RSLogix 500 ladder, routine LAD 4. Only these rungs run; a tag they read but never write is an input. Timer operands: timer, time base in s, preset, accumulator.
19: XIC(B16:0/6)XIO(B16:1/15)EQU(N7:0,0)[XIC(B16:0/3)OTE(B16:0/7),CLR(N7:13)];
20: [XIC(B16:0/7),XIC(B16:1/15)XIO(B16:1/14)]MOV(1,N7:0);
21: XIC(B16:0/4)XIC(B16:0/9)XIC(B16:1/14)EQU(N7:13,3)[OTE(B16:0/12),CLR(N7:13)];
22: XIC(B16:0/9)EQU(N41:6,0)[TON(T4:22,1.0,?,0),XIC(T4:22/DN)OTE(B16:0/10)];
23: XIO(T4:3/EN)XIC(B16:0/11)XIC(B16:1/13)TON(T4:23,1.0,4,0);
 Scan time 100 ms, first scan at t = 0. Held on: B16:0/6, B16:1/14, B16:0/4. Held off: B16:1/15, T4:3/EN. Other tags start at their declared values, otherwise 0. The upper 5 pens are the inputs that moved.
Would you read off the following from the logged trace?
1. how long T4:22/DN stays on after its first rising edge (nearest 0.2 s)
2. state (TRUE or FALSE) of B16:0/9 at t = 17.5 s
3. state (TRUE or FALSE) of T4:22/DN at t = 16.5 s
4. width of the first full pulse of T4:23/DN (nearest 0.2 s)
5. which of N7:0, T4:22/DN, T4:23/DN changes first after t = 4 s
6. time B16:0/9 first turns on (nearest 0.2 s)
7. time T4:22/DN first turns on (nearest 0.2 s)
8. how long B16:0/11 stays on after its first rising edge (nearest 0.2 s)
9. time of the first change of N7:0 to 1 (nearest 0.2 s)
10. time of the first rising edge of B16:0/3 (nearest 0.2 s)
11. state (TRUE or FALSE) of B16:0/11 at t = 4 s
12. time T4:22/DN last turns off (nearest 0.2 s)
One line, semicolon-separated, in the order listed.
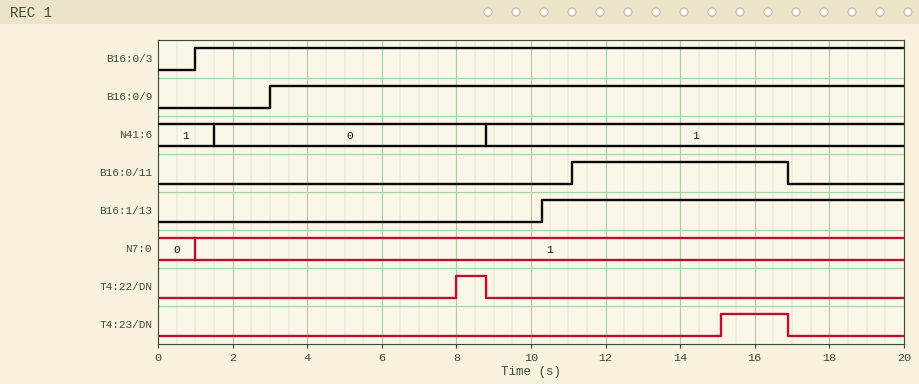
0.8 s; TRUE; FALSE; 1.8 s; T4:22/DN; 3.0 s; 8.0 s; 5.8 s; 1.0 s; 1.0 s; FALSE; 8.8 s
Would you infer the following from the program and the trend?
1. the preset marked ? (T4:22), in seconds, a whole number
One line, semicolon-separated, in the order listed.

5 s
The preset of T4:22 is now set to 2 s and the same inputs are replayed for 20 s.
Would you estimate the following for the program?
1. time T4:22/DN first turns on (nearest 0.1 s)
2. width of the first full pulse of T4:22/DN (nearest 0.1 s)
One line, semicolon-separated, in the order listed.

5.0 s; 3.8 s
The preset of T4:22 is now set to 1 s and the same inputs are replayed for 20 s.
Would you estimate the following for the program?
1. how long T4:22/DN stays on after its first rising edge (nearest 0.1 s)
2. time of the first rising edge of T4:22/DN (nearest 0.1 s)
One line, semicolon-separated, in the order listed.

4.8 s; 4.0 s
